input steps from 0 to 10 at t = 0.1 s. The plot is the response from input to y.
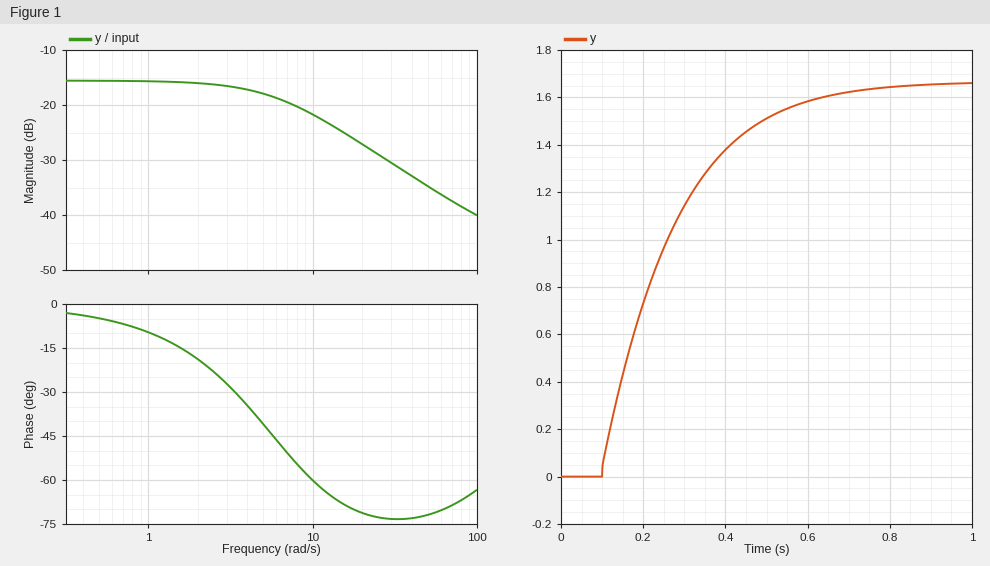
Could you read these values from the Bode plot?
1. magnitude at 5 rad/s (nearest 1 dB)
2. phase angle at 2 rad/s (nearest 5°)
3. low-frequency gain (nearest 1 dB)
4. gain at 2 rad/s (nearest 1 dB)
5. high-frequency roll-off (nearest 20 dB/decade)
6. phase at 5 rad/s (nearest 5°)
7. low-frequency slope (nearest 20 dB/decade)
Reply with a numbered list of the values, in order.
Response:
1. -18 dB
2. -20°
3. -16 dB
4. -16 dB
5. -20 dB/decade
6. -40°
7. 0 dB/decade
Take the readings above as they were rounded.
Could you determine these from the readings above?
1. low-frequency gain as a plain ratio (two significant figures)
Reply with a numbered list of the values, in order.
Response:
1. 0.16
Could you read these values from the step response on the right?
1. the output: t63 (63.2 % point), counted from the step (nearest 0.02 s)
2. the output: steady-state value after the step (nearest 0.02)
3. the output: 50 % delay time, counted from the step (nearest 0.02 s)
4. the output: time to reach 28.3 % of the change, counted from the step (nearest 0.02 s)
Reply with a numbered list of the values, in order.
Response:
1. 0.18 s
2. 1.66
3. 0.12 s
4. 0.06 s
